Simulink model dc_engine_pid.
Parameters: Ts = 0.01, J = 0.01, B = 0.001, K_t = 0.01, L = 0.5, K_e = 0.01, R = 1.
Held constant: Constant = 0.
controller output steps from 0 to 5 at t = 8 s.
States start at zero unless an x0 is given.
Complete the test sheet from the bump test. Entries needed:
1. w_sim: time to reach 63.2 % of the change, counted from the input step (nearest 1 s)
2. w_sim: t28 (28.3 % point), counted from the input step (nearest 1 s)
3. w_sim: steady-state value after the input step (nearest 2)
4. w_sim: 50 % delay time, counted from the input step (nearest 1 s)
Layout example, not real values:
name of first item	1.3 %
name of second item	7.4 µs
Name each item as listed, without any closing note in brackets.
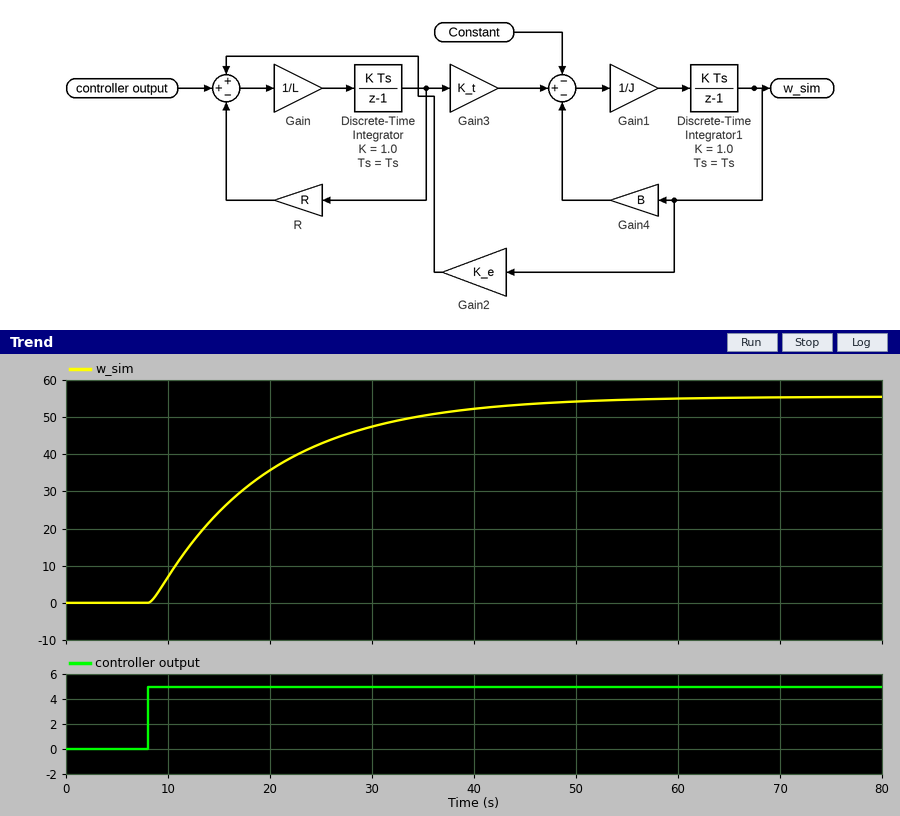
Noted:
w_sim: time to reach 63.2 % of the change, counted from the input step	12 s
w_sim: t28 (28.3 % point), counted from the input step	4 s
w_sim: steady-state value after the input step	56
w_sim: 50 % delay time, counted from the input step	8 s
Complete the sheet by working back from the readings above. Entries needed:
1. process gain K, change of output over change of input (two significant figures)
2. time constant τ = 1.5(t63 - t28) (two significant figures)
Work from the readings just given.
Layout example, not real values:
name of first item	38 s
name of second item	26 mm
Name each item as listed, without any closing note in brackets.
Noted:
process gain K, change of output over change of input	11
time constant τ = 1.5(t63 - t28)	12 s
